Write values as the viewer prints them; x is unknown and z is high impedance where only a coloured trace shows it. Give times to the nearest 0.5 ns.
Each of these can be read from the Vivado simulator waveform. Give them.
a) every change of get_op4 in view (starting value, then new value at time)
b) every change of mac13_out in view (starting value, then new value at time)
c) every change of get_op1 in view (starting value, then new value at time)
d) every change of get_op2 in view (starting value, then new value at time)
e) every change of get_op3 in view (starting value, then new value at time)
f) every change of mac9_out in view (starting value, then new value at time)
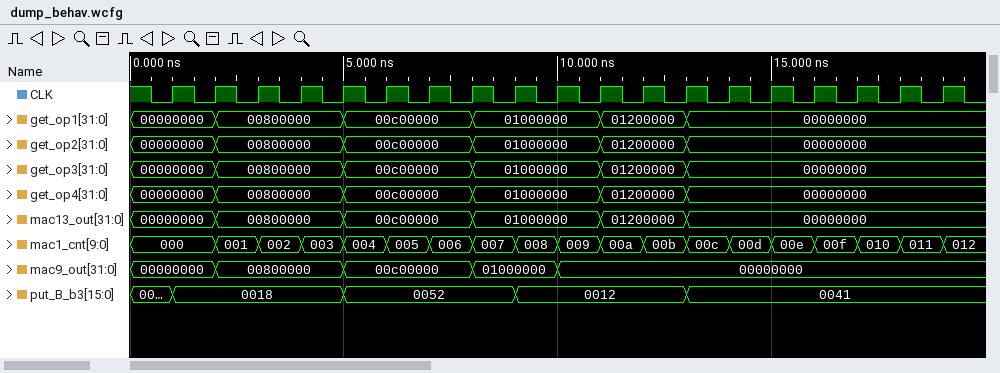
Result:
00000000, 00800000 at 2 ns, 00c00000 at 5 ns, 01000000 at 8 ns, 01200000 at 11 ns, 00000000 at 13 ns
00000000, 00800000 at 2 ns, 00c00000 at 5 ns, 01000000 at 8 ns, 01200000 at 11 ns, 00000000 at 13 ns
00000000, 00800000 at 2 ns, 00c00000 at 5 ns, 01000000 at 8 ns, 01200000 at 11 ns, 00000000 at 13 ns
00000000, 00800000 at 2 ns, 00c00000 at 5 ns, 01000000 at 8 ns, 01200000 at 11 ns, 00000000 at 13 ns
00000000, 00800000 at 2 ns, 00c00000 at 5 ns, 01000000 at 8 ns, 01200000 at 11 ns, 00000000 at 13 ns
00000000, 00800000 at 2 ns, 00c00000 at 5 ns, 01000000 at 8 ns, 00000000 at 10 ns
